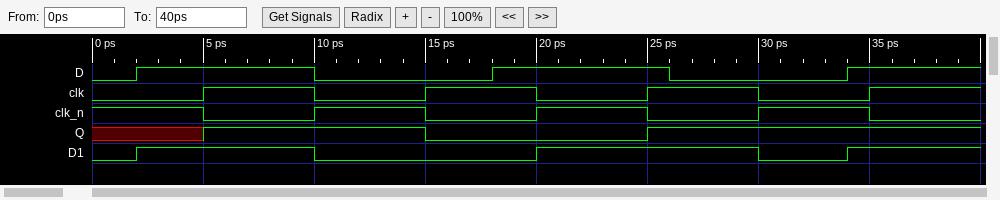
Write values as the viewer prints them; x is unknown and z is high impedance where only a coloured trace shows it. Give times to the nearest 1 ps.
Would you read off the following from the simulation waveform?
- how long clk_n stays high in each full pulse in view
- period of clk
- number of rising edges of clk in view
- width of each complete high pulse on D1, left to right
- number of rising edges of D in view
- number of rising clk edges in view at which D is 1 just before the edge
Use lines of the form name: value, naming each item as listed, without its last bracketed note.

how long clk_n stays high in each full pulse in view: 5 ps, 5 ps, 5 ps
period of clk: 10 ps
number of rising edges of clk in view: 4
width of each complete high pulse on D1, left to right: 8 ps, 10 ps
number of rising edges of D in view: 3
number of rising clk edges in view at which D is 1 just before the edge: 3
